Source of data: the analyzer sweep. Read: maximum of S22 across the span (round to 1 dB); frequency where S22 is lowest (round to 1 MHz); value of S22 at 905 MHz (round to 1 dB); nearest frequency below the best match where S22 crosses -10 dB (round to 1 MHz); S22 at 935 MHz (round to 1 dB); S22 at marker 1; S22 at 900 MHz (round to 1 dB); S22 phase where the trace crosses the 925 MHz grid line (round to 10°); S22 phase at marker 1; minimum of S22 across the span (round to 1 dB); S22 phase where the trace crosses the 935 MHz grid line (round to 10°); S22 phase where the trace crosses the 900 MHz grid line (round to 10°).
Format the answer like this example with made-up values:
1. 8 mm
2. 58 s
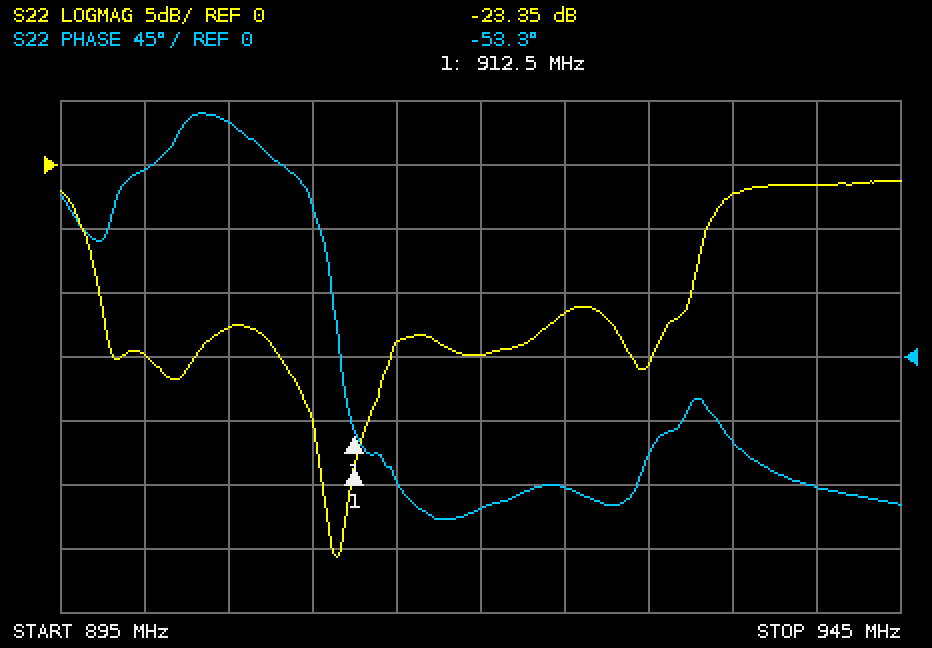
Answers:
1. -1 dB
2. 911 MHz
3. -13 dB
4. 897 MHz
5. -2 dB
6. -23.35 dB
7. -15 dB
8. -90°
9. -53.3°
10. -31 dB
11. -60°
12. 130°
